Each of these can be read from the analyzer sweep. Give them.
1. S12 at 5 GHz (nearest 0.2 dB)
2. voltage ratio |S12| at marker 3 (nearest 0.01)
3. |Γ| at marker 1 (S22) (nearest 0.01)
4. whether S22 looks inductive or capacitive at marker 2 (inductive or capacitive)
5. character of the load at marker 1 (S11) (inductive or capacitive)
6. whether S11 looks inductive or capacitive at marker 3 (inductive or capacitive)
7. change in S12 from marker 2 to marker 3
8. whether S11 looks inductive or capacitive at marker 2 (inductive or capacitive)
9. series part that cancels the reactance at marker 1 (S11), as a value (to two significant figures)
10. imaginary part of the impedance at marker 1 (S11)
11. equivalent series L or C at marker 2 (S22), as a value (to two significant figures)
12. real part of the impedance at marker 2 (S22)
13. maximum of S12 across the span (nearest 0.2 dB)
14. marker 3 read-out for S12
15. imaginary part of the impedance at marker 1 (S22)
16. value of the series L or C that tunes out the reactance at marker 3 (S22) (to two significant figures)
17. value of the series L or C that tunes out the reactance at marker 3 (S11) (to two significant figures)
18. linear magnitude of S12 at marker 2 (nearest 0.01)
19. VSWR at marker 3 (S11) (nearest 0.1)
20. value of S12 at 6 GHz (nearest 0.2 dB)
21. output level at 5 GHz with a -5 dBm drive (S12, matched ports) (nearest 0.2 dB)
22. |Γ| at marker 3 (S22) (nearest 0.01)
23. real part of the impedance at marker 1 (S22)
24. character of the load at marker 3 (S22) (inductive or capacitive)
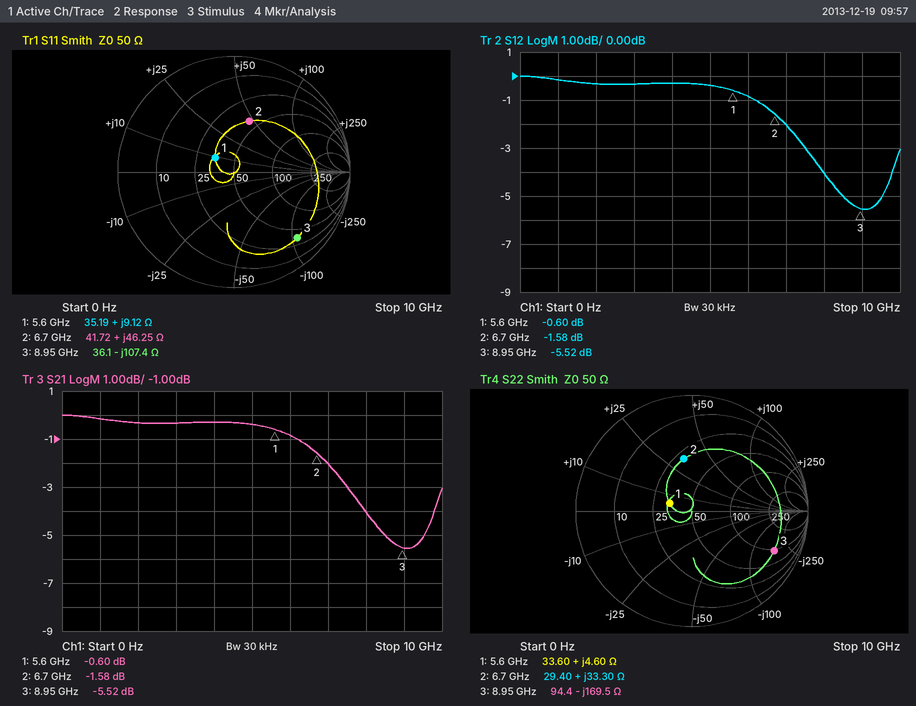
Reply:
-0.4 dB
0.53
0.20
inductive
inductive
capacitive
-3.94 dB
inductive
3.1 pF
+9.12 Ω
790 pH
29.40 Ω
0.0 dB
-5.52 dB
+4.60 Ω
3.0 nH
1.9 nH
0.83
8.4
-0.8 dB
-5.4 dBm
0.79
33.60 Ω
capacitive
